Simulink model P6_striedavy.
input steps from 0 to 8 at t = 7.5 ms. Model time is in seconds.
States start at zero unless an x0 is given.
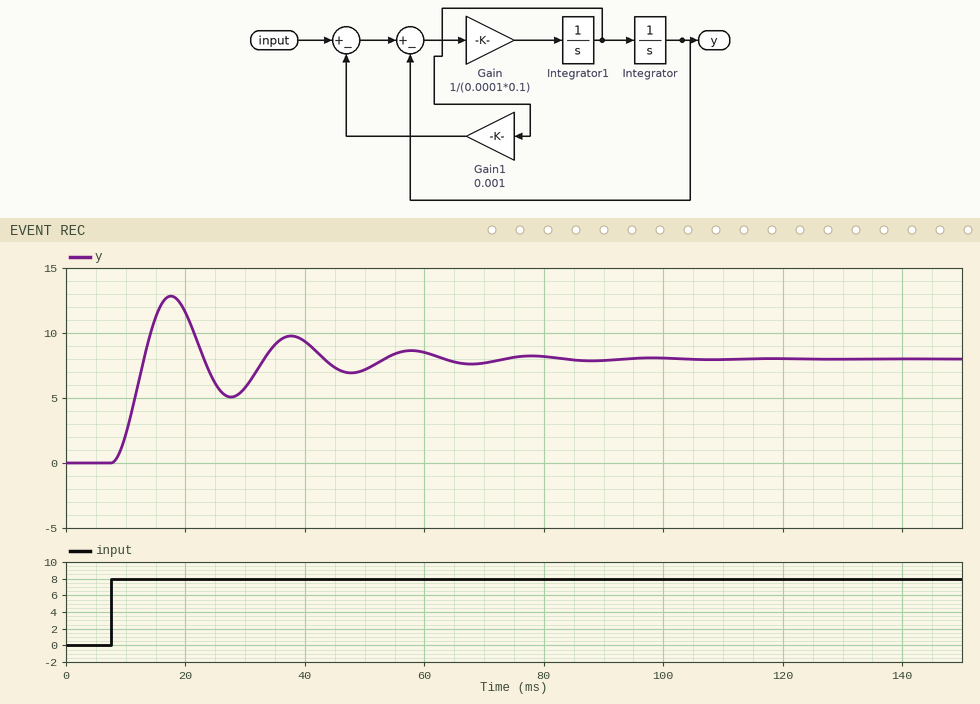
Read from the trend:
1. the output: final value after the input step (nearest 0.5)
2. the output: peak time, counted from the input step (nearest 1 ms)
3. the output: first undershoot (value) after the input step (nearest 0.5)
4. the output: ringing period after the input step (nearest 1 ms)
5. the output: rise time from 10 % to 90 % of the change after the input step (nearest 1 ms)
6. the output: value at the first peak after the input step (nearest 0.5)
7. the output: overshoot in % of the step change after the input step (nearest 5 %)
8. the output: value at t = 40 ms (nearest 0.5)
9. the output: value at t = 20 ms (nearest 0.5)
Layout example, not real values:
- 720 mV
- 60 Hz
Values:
- 8.0
- 10 ms
- 5.0
- 20 ms
- 4 ms
- 13.0
- 60 %
- 9.5
- 11.5
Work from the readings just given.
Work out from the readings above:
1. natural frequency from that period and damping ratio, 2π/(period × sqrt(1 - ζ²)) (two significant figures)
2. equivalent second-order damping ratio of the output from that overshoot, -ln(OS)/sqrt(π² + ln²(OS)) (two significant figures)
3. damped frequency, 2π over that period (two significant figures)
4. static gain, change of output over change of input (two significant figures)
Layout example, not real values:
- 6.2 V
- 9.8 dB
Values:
- 0.32 rad/ms
- 0.16
- 0.31 rad/ms
- 1.0
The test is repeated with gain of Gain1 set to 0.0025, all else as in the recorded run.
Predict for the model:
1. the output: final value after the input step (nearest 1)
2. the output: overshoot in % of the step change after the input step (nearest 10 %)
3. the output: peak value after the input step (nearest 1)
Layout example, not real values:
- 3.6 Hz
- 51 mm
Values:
- 8
- 30 %
- 10
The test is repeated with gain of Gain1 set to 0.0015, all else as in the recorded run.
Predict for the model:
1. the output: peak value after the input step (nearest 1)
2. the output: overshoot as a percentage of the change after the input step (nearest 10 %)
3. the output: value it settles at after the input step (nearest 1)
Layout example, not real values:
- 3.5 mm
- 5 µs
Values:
- 12
- 50 %
- 8
